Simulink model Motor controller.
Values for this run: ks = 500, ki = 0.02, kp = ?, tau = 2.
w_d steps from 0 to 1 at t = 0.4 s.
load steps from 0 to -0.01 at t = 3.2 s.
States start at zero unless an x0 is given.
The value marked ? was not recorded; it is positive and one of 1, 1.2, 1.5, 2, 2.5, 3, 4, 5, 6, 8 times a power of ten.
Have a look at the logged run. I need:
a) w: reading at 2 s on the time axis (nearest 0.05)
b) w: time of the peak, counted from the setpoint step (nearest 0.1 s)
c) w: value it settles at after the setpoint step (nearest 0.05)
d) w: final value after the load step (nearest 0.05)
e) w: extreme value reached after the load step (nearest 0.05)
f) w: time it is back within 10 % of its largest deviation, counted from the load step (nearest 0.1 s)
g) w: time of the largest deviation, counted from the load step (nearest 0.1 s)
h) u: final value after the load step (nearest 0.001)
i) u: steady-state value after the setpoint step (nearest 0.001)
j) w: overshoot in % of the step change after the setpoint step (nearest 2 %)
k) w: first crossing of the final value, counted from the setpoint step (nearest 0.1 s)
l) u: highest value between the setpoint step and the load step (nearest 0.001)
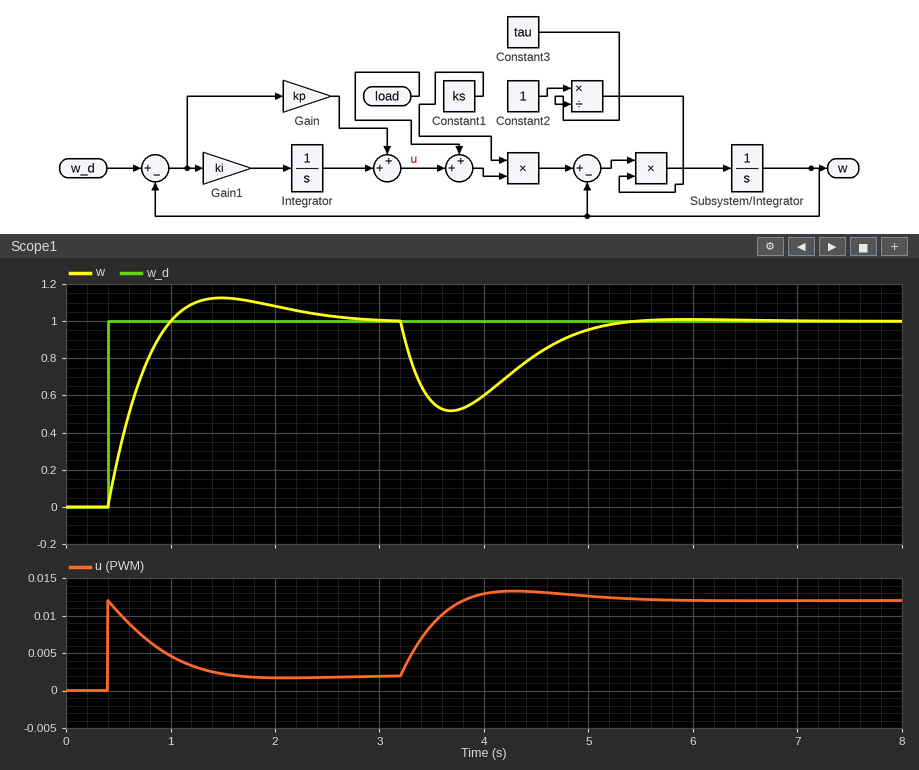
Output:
1.10
1.1 s
1.00
1.00
0.50
1.8 s
0.5 s
0.012
0.002
12 %
0.6 s
0.012
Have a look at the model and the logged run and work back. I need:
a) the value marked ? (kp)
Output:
0.012
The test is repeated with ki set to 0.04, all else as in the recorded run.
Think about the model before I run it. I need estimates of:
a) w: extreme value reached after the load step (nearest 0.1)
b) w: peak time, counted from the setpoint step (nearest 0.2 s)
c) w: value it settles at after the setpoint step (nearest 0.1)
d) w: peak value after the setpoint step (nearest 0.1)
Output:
0.6
0.8 s
1.0
1.2
